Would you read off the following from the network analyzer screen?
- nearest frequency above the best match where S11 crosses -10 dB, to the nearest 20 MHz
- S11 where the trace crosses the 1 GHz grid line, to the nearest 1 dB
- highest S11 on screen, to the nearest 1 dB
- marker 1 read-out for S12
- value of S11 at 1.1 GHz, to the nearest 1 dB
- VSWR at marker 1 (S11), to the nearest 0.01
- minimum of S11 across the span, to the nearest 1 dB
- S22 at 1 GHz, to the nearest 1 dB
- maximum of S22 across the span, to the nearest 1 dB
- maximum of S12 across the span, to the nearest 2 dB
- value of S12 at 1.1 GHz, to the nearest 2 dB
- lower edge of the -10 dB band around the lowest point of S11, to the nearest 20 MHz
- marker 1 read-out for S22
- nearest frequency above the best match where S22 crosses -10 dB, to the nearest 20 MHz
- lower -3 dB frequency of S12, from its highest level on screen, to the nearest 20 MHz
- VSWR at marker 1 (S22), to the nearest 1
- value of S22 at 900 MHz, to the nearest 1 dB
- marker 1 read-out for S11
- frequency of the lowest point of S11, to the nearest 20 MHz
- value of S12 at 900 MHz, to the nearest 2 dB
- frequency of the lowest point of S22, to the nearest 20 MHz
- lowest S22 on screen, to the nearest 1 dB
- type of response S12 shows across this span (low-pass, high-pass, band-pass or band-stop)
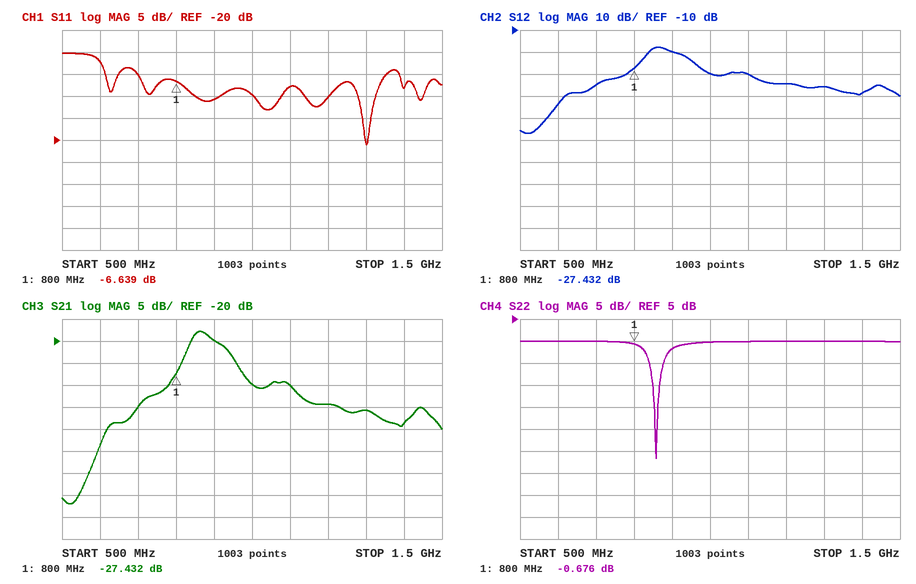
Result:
1.32 GHz
-10 dB
0 dB
-27.432 dB
-8 dB
2.74
-21 dB
0 dB
0 dB
-18 dB
-30 dB
1.28 GHz
-0.676 dB
860 MHz
840 MHz
26
-2 dB
-6.639 dB
1.30 GHz
-20 dB
860 MHz
-27 dB
band-pass
